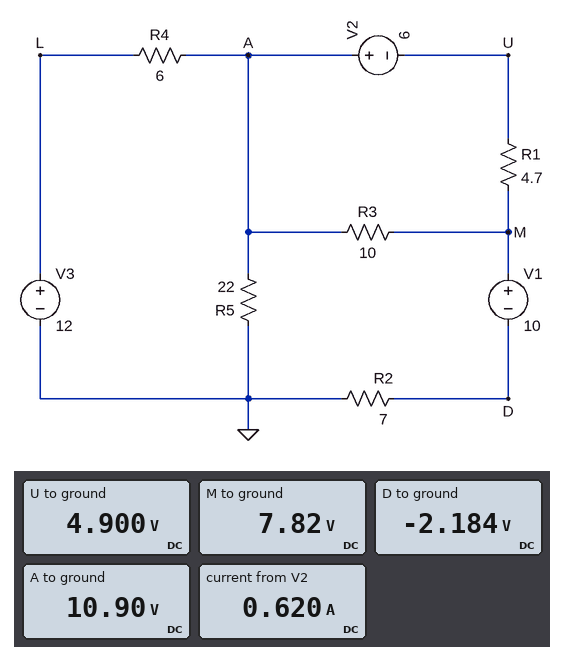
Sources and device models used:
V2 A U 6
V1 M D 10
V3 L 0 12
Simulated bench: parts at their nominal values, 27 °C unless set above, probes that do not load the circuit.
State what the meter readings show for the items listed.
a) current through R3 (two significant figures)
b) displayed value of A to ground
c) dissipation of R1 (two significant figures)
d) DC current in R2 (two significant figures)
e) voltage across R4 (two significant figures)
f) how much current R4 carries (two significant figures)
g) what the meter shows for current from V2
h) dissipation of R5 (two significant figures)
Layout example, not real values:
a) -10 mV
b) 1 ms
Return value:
a) 310 mA
b) 10.90 V
c) 1.8 W
d) 310 mA
e) 1.1 V
f) 180 mA
g) 0.620 A
h) 5.4 W
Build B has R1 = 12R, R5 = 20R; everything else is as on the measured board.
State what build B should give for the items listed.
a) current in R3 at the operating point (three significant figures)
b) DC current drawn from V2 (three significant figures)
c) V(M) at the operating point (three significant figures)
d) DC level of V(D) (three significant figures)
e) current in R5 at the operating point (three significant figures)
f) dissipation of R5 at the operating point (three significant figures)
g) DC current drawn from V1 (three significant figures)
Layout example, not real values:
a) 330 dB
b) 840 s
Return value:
a) 161 mA
b) 366 mA
c) 8.57 V
d) -1.43 V
e) 509 mA
f) 5.18 W
g) 205 mA
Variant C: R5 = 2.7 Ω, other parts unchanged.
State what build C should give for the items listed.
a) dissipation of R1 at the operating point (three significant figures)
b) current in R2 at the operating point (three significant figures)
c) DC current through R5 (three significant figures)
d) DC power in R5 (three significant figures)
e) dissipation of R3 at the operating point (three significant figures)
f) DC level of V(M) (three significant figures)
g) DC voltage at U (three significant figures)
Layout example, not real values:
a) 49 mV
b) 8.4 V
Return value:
a) 4.63 W
b) 859 mA
c) 1.97 A
d) 10.5 W
e) 178 mW
f) 3.99 V
g) -677 mV
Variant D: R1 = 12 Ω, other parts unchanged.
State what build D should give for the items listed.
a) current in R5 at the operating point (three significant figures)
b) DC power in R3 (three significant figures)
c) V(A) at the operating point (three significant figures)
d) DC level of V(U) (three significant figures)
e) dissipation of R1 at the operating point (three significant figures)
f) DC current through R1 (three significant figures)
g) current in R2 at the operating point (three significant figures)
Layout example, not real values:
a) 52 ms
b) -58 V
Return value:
a) 470 mA
b) 282 mW
c) 10.3 V
d) 4.33 V
e) 1.56 W
f) 360 mA
g) 192 mA
